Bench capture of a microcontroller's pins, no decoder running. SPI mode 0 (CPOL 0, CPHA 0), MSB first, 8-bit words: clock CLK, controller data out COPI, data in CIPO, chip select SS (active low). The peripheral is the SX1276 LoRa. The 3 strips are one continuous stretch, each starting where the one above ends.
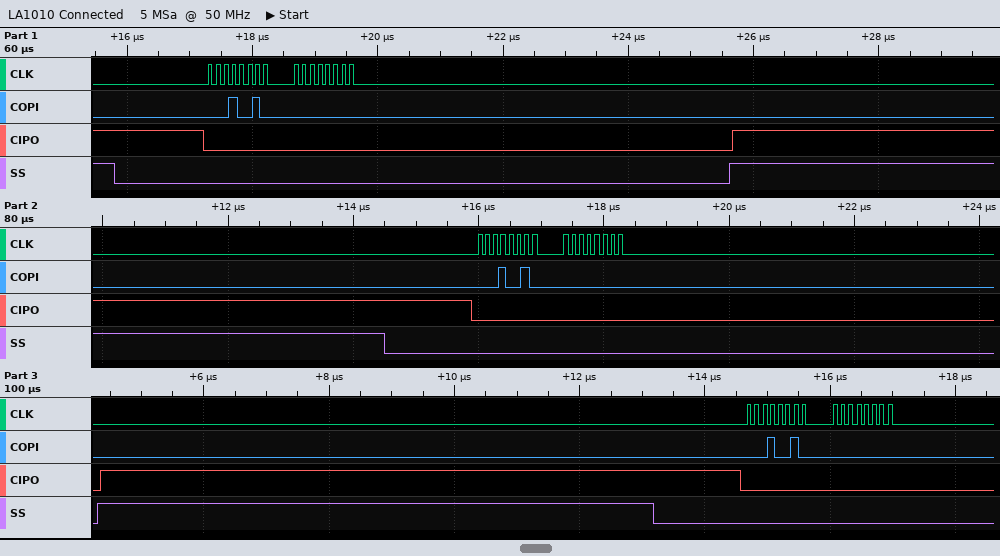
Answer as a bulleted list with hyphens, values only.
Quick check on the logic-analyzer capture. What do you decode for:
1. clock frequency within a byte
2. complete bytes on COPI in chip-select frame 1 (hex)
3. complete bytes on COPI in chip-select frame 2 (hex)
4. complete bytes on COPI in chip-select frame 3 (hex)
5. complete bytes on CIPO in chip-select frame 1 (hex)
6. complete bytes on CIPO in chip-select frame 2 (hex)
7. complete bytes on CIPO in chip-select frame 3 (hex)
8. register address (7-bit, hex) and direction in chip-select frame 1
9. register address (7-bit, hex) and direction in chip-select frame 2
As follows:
- 8 MHz
- 0x12 0x00
- 0x12 0x00
- 0x12 0x00
- 0x00 0x00
- 0x00 0x00
- 0x00 0x00
- 0x12 read
- 0x12 read
